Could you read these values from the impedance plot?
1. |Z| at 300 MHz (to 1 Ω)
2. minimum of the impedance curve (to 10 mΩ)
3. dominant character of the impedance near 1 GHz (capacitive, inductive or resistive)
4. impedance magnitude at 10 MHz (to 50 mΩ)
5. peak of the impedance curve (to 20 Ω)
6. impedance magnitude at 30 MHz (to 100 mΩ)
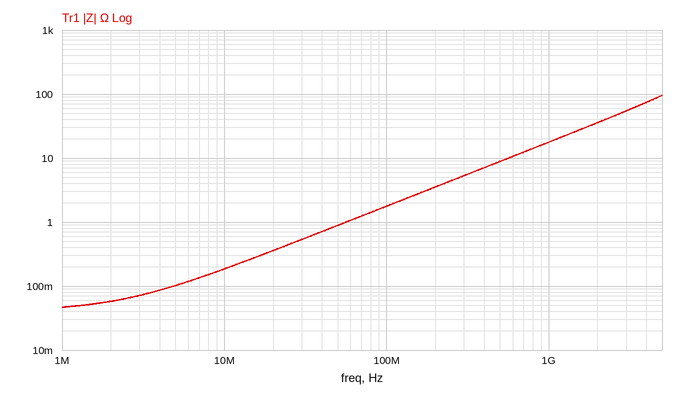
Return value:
5 Ω
50 mΩ
inductive
200 mΩ
100 Ω
500 mΩ
